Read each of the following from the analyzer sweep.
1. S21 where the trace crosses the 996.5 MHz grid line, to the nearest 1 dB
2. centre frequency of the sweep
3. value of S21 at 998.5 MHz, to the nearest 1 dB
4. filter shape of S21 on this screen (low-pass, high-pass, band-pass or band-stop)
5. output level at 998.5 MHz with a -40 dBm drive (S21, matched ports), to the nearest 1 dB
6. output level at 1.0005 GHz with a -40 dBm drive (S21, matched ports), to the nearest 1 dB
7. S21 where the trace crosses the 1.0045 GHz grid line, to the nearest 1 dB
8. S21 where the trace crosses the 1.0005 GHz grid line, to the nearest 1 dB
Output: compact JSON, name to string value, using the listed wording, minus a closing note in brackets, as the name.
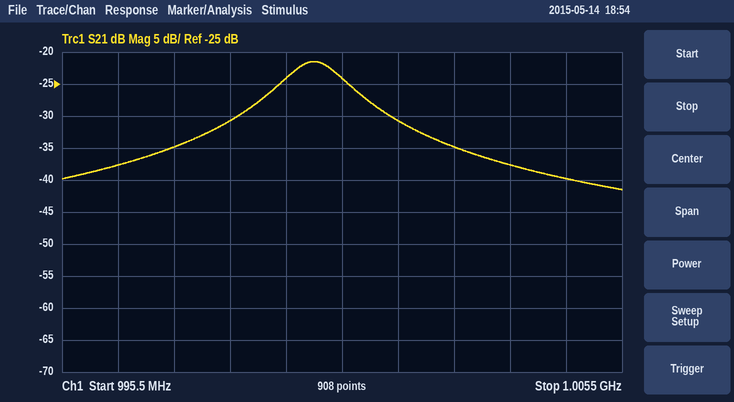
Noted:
{"S21 where the trace crosses the 996.5 MHz grid line, to the nearest 1 dB": "-38 dB", "centre frequency of the sweep": "1.0005 GHz", "value of S21 at 998.5 MHz, to the nearest 1 dB": "-31 dB", "filter shape of S21 on this screen": "band-pass", "output level at 998.5 MHz with a -40 dBm drive (S21, matched ports), to the nearest 1 dB": "-71 dBm", "output level at 1.0005 GHz with a -40 dBm drive (S21, matched ports), to the nearest 1 dB": "-64 dBm", "S21 where the trace crosses the 1.0045 GHz grid line, to the nearest 1 dB": "-40 dB", "S21 where the trace crosses the 1.0005 GHz grid line, to the nearest 1 dB": "-24 dB"}
